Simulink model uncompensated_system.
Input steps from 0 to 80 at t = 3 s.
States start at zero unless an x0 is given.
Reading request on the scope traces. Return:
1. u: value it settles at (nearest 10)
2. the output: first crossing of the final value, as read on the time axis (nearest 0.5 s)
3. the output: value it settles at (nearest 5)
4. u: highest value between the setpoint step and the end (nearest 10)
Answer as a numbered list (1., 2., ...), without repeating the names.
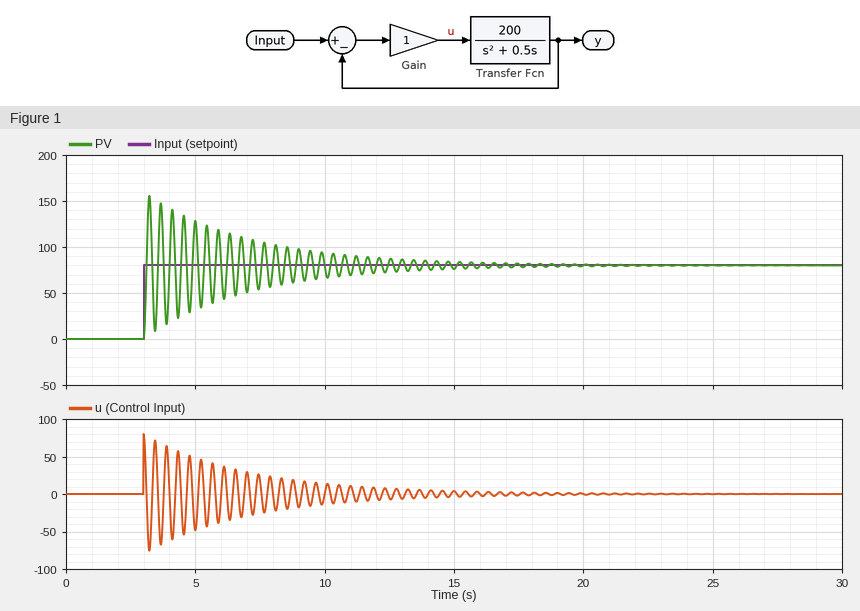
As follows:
1. 0
2. 3.0 s
3. 80
4. 80
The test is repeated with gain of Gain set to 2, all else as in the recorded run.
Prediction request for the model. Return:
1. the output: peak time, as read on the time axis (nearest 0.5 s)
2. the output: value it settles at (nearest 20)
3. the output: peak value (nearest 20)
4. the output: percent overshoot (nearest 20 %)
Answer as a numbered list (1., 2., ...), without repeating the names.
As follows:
1. 3.0 s
2. 80
3. 160
4. 100 %
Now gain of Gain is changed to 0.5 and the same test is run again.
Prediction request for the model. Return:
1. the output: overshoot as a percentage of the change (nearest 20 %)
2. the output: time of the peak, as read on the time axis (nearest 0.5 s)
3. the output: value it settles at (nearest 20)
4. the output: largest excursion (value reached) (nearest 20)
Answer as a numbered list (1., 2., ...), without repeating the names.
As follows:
1. 100 %
2. 3.5 s
3. 80
4. 160
